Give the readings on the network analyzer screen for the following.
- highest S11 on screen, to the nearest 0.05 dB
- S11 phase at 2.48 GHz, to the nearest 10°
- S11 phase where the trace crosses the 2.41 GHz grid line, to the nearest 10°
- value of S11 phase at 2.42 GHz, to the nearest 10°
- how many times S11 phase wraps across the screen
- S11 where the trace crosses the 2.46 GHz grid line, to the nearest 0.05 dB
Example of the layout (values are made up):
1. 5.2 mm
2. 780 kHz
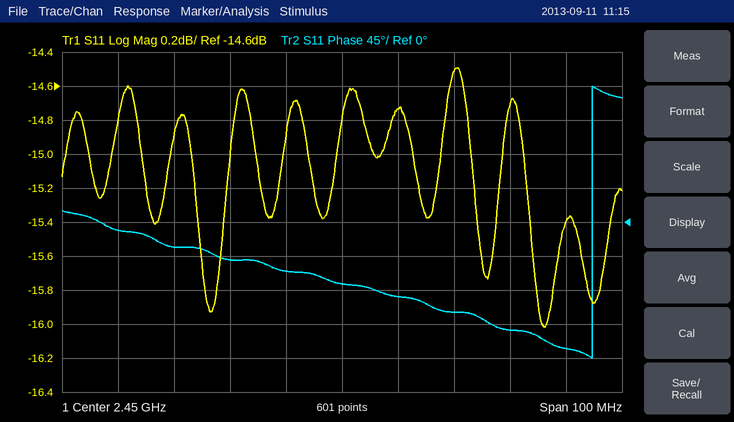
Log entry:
1. -14.50 dB
2. -140°
3. -10°
4. -30°
5. 1
6. -14.75 dB
